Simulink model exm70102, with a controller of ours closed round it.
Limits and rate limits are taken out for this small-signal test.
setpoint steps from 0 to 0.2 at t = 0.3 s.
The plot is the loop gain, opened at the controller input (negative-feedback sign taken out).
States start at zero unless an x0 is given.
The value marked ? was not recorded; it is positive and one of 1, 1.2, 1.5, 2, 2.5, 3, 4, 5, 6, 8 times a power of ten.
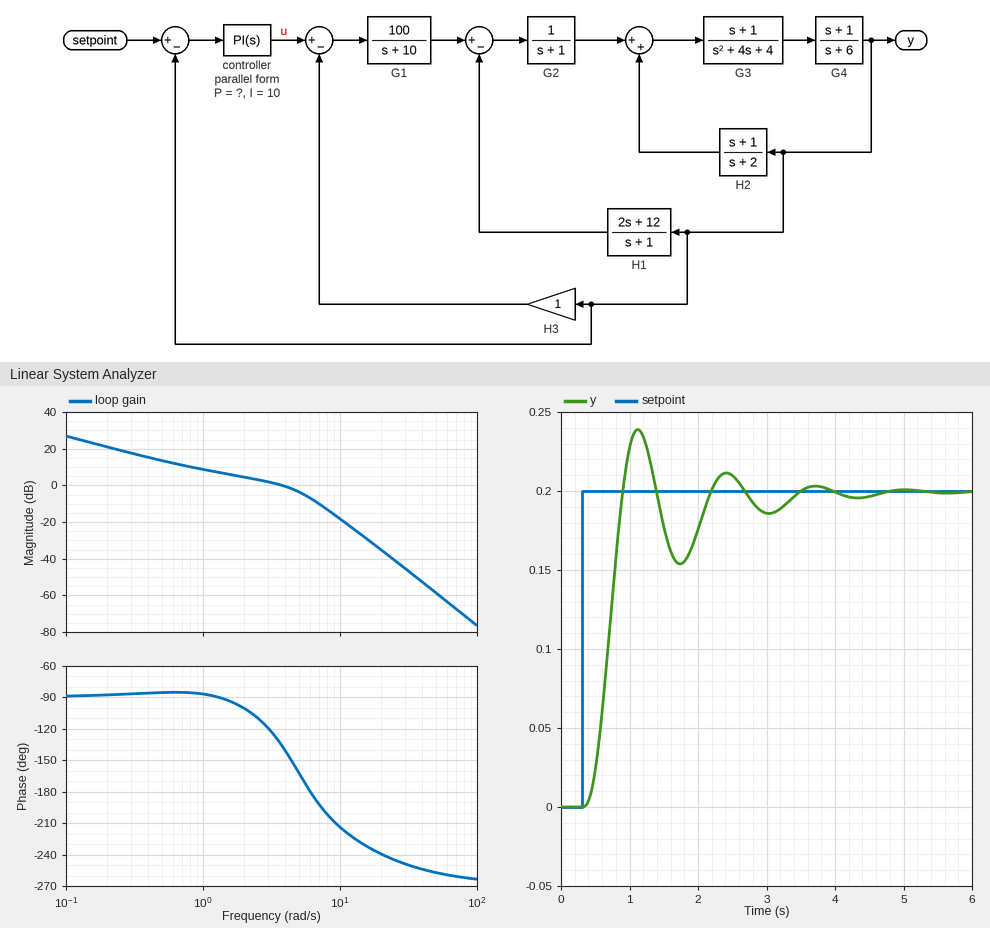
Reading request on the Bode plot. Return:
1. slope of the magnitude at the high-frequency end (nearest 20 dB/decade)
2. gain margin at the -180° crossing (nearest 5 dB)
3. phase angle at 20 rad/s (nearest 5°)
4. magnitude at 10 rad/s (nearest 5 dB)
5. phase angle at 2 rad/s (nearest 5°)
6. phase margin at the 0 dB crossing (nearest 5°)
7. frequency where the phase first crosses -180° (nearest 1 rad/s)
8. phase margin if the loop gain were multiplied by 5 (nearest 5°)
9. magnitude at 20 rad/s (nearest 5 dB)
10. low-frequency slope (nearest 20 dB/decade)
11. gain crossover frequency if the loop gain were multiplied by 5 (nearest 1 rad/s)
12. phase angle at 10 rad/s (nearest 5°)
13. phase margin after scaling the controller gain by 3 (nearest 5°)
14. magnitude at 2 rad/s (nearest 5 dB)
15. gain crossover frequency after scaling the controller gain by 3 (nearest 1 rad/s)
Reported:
-60 dB/decade
5 dB
-240°
-20 dB
-100°
45°
6 rad/s
-25°
-35 dB
-20 dB/decade
8 rad/s
-215°
-10°
5 dB
7 rad/s
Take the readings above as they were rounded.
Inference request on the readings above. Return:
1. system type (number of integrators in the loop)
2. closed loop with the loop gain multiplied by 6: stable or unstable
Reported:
1
unstable
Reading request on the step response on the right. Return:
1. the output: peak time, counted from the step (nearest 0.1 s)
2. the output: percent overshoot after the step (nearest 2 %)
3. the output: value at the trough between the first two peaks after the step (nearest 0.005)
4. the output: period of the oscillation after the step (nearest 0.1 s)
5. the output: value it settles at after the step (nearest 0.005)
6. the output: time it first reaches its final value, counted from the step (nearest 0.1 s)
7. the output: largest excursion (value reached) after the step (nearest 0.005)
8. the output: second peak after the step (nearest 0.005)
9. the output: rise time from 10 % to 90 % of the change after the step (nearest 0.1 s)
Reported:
0.8 s
20 %
0.155
1.3 s
0.200
0.6 s
0.240
0.210
0.4 s
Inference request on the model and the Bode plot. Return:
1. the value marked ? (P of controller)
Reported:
1.5
